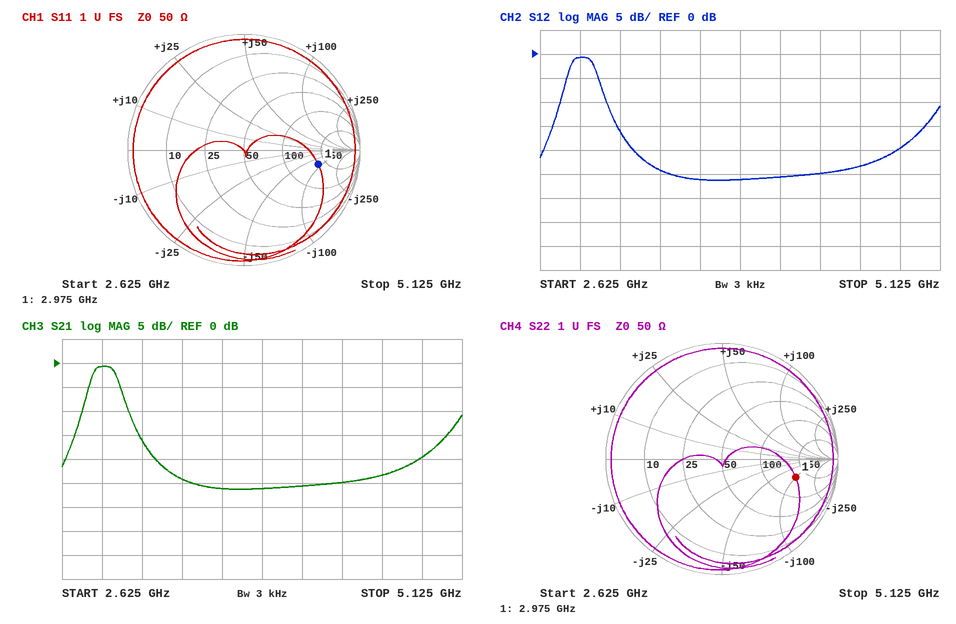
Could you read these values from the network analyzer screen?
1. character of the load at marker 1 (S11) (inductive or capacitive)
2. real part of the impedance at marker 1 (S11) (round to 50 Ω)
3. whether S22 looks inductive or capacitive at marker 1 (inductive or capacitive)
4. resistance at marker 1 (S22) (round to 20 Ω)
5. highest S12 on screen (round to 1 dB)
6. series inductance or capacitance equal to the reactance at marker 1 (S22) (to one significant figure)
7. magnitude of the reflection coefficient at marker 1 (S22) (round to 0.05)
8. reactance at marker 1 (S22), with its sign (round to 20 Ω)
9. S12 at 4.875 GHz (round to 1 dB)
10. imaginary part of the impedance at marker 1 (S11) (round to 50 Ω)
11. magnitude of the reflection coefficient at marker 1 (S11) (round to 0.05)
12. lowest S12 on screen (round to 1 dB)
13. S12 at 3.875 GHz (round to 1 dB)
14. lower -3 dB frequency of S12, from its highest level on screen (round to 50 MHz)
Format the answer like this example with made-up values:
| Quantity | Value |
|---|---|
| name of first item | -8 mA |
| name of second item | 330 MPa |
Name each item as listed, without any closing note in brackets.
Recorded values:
| Quantity | Value |
|---|---|
| character of the load at marker 1 (S11) | capacitive |
| real part of the impedance at marker 1 (S11) | 200 Ω |
| whether S22 looks inductive or capacitive at marker 1 | capacitive |
| resistance at marker 1 (S22) | 180 Ω |
| highest S12 on screen | -1 dB |
| series inductance or capacitance equal to the reactance at marker 1 (S22) | 500 fF |
| magnitude of the reflection coefficient at marker 1 (S22) | 0.65 |
| reactance at marker 1 (S22), with its sign | -100 Ω |
| S12 at 4.875 GHz | -20 dB |
| imaginary part of the impedance at marker 1 (S11) | -100 Ω |
| magnitude of the reflection coefficient at marker 1 (S11) | 0.65 |
| lowest S12 on screen | -26 dB |
| S12 at 3.875 GHz | -26 dB |
| lower -3 dB frequency of S12, from its highest level on screen | 2.80 GHz |
